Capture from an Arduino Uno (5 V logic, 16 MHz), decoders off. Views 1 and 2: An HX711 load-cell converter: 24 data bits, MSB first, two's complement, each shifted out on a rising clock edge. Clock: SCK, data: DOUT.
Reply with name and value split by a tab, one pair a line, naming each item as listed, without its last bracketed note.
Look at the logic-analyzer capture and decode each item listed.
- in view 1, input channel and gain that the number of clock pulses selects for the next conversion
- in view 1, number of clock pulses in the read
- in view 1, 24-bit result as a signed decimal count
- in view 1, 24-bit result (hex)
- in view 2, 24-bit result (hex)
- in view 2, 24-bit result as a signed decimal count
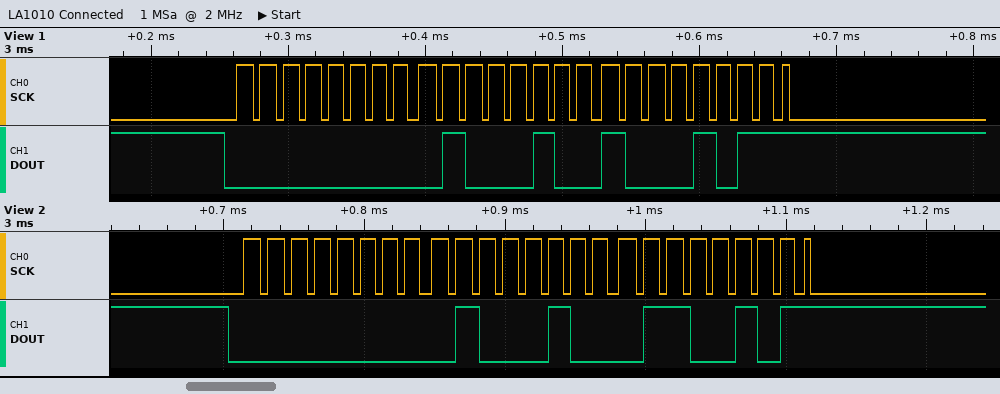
in view 1, input channel and gain that the number of clock pulses selects for the next conversion	channel A, gain 128
in view 1, number of clock pulses in the read	25
in view 1, 24-bit result as a signed decimal count	17547
in view 1, 24-bit result	0x00448B
in view 2, 24-bit result	0x004465
in view 2, 24-bit result as a signed decimal count	17509
